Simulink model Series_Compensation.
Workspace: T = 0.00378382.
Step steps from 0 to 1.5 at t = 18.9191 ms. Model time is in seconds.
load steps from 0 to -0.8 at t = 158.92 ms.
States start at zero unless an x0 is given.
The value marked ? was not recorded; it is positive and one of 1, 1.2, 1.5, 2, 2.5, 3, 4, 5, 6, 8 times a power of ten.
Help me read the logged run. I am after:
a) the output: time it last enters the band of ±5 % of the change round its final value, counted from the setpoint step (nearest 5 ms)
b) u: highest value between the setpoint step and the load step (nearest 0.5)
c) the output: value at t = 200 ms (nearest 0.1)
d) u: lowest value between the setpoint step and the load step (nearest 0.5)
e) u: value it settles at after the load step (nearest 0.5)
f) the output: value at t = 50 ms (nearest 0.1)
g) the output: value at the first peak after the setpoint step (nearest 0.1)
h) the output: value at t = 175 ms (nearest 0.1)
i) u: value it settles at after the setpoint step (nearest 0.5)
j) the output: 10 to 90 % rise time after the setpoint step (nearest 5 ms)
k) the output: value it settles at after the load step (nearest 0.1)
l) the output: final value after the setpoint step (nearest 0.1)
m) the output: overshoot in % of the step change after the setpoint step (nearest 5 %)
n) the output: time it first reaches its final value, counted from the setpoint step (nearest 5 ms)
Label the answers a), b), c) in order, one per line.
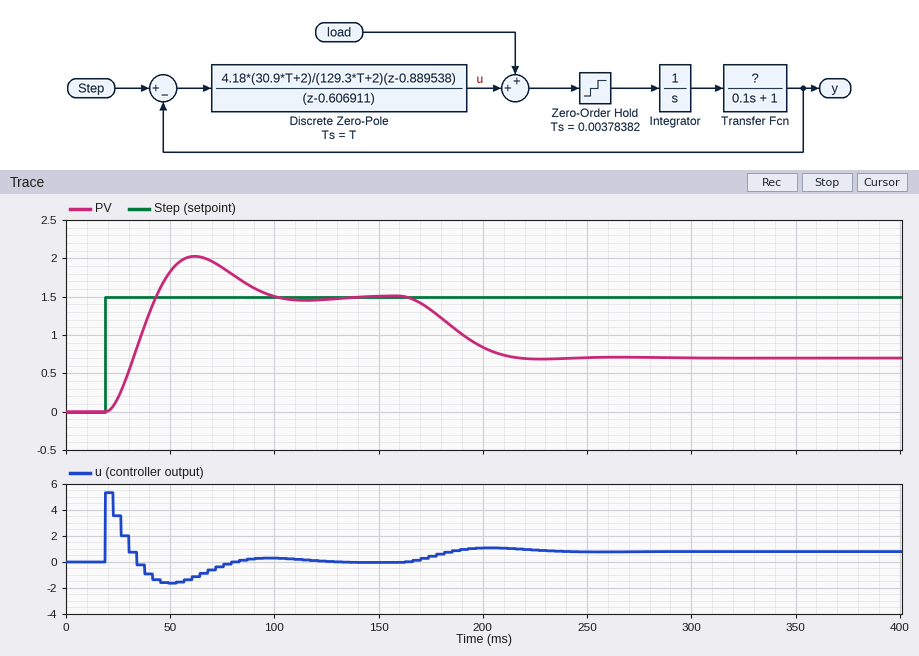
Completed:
a) 75 ms
b) 5.5
c) 0.8
d) -1.5
e) 1.0
f) 1.8
g) 2.0
h) 1.3
i) 0.0
j) 15 ms
k) 0.7
l) 1.5
m) 35 %
n) 25 ms
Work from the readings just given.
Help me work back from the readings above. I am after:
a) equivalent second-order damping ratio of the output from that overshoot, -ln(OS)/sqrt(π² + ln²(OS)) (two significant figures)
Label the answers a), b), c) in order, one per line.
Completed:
a) 0.32
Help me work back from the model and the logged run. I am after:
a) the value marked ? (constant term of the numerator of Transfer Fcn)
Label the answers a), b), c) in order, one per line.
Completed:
a) 200
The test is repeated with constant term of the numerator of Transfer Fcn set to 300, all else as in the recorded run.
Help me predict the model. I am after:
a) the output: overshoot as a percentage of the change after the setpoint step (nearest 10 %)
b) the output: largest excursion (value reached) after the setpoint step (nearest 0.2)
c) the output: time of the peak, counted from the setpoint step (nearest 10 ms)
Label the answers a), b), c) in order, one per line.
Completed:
a) 40 %
b) 2.2
c) 30 ms
